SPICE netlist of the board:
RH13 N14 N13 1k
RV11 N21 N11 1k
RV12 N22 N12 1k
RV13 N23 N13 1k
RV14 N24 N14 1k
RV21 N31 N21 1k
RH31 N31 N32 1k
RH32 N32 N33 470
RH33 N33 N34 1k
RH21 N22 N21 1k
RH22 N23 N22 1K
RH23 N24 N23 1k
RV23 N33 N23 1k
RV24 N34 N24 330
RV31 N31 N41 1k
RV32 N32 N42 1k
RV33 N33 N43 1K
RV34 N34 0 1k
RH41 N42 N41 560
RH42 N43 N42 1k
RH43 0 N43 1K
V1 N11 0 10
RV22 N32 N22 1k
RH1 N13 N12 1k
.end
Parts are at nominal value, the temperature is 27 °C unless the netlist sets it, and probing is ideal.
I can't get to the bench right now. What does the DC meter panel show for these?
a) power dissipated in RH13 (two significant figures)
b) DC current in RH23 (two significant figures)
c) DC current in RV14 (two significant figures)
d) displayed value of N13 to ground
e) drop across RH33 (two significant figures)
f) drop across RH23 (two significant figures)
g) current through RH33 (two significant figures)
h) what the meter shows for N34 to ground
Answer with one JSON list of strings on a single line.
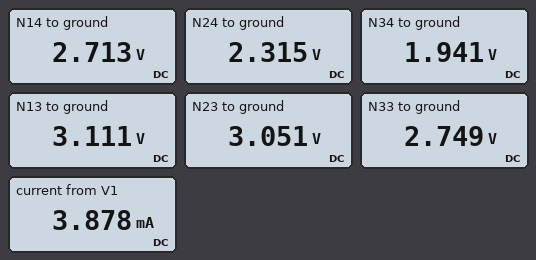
["160 µW", "740 µA", "400 µA", "3.111 V", "810 mV", "740 mV", "810 µA", "1.941 V"]
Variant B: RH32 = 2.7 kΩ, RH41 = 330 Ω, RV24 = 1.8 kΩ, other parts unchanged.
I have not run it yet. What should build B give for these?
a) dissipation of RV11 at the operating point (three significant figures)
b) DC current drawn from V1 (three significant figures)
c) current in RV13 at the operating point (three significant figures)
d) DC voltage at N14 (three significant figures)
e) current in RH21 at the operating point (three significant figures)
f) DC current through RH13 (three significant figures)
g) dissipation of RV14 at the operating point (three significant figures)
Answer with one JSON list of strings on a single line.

["13.0 mW", "3.61 mA", "167 µA", "3.21 V", "1.96 mA", "296 µA", "87.8 µW"]
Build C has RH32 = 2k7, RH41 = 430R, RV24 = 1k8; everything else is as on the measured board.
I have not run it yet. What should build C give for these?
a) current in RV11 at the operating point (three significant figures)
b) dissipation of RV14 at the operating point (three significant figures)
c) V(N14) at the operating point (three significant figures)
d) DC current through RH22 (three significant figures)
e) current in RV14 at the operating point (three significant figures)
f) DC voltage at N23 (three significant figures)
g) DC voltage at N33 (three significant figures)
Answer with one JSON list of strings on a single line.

["3.60 mA", "88.0 µW", "3.21 V", "1.10 mA", "297 µA", "3.34 V", "2.50 V"]
